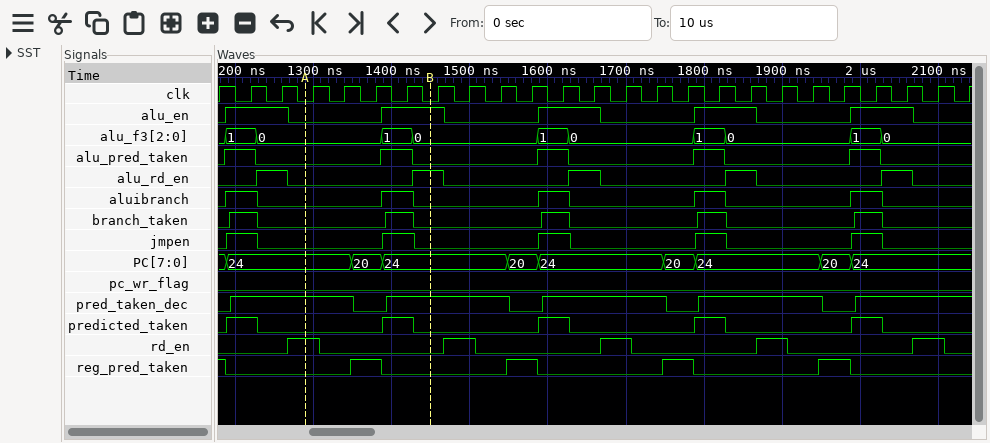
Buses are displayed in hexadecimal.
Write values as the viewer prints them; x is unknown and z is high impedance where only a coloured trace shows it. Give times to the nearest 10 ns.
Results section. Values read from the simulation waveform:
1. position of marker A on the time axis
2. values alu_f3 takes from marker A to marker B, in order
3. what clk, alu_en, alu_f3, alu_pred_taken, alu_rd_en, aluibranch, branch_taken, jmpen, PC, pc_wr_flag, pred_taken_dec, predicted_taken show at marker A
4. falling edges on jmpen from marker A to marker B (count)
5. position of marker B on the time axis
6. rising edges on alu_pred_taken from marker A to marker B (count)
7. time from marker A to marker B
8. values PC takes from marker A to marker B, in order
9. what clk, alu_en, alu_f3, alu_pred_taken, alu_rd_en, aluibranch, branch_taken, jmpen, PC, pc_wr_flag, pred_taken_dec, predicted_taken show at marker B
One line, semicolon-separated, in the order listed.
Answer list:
1290 ns; 0, 1, 0; clk=0, alu_en=0, alu_f3=0, alu_pred_taken=0, alu_rd_en=0, aluibranch=0, branch_taken=0, jmpen=0, PC=24, pc_wr_flag=0, pred_taken_dec=1, predicted_taken=0; 1; 1450 ns; 1; 160 ns; 24, 20, 24; clk=0, alu_en=1, alu_f3=0, alu_pred_taken=0, alu_rd_en=1, aluibranch=0, branch_taken=0, jmpen=0, PC=24, pc_wr_flag=0, pred_taken_dec=1, predicted_taken=0
